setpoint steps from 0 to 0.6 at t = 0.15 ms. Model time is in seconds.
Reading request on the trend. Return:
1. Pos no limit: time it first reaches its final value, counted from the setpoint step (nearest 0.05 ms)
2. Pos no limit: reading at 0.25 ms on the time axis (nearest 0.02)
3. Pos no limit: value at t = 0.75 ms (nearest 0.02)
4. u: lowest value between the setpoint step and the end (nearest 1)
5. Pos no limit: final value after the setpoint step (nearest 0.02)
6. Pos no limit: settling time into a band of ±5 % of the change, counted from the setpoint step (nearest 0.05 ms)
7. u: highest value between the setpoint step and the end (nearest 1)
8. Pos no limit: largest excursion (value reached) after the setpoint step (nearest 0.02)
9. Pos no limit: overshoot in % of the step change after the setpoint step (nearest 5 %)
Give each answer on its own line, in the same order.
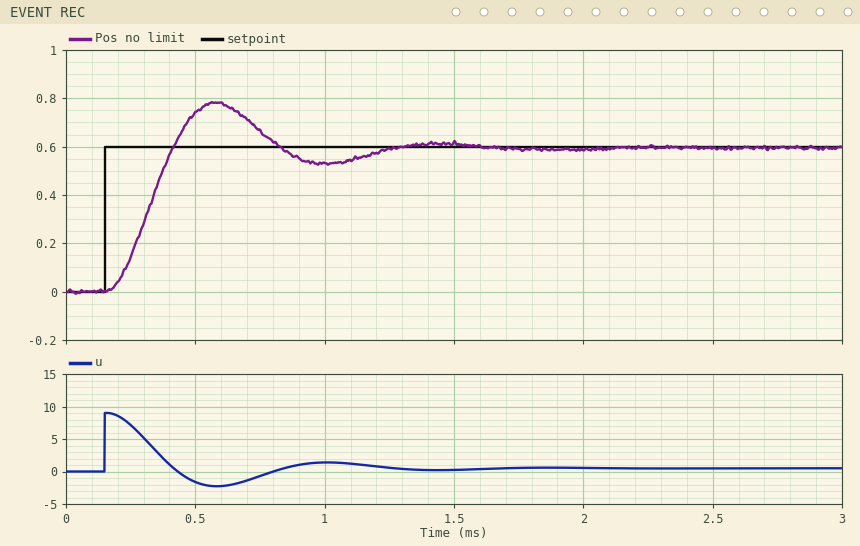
0.25 ms
0.14
0.66
-2
0.60
1.05 ms
9
0.78
30 %
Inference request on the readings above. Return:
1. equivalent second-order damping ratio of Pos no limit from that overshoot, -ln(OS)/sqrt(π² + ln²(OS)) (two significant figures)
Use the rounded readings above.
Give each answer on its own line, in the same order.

0.36
